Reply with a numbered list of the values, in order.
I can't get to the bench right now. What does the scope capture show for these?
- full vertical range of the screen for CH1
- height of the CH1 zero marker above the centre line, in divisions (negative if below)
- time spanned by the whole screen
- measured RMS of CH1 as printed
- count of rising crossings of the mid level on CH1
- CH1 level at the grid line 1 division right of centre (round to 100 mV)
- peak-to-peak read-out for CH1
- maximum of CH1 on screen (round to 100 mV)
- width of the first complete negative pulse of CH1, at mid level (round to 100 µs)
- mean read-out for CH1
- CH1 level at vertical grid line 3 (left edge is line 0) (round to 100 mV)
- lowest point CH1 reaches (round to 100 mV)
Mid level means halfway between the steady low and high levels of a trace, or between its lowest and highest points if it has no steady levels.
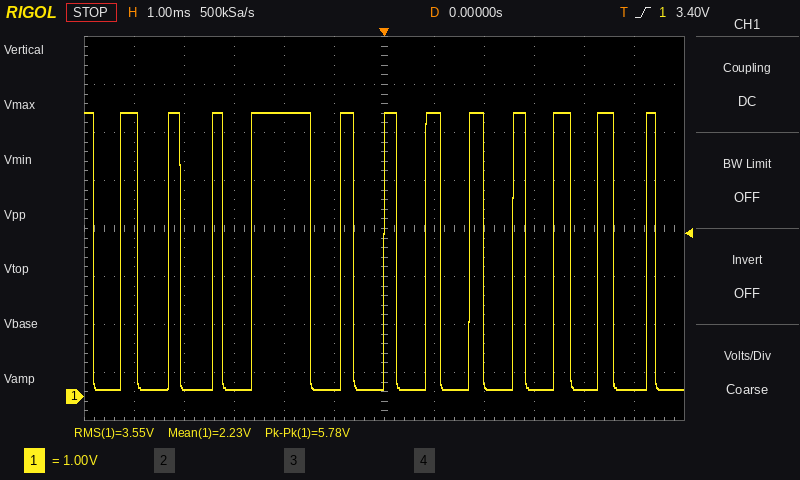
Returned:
1. 8 V
2. -3.5 div
3. 12 ms
4. 3.55 V
5. 12
6. 5.9 V
7. 5.78 V
8. 5.9 V
9. 500 µs
10. 2.23 V
11. 100 mV
12. 100 mV
